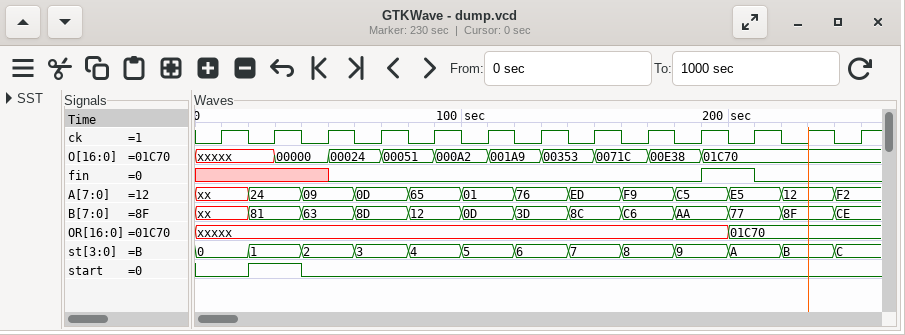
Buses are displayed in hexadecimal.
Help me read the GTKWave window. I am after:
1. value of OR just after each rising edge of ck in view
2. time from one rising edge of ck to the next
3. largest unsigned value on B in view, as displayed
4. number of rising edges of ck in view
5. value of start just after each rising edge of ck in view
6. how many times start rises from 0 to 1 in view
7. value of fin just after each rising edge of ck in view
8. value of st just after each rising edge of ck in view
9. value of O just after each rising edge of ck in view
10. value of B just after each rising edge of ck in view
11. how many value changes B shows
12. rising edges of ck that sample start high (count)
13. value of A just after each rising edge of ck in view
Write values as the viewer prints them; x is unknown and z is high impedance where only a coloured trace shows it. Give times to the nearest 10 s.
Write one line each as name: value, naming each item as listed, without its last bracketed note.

value of OR just after each rising edge of ck in view: xxxxx, xxxxx, xxxxx, xxxxx, xxxxx, xxxxx, xxxxx, xxxxx, xxxxx, xxxxx, 01C70, 01C70, 01C70
time from one rising edge of ck to the next: 20 s
largest unsigned value on B in view, as displayed: CE
number of rising edges of ck in view: 13
value of start just after each rising edge of ck in view: 0 1 0 0 0 0 0 0 0 0 0 0 0
how many times start rises from 0 to 1 in view: 1
value of fin just after each rising edge of ck in view: x x 0 0 0 0 0 0 0 1 0 0 0
value of st just after each rising edge of ck in view: 0, 1, 2, 3, 4, 5, 6, 7, 8, 9, A, B, C
value of O just after each rising edge of ck in view: xxxxx, 00000, 00024, 00051, 000A2, 001A9, 00353, 0071C, 00E38, 01C70, 01C70, 01C70, 01C70
value of B just after each rising edge of ck in view: xx, 81, 63, 8D, 12, 0D, 3D, 8C, C6, AA, 77, 8F, CE
how many value changes B shows: 12
rising edges of ck that sample start high: 1
value of A just after each rising edge of ck in view: xx, 24, 09, 0D, 65, 01, 76, ED, F9, C5, E5, 12, F2
